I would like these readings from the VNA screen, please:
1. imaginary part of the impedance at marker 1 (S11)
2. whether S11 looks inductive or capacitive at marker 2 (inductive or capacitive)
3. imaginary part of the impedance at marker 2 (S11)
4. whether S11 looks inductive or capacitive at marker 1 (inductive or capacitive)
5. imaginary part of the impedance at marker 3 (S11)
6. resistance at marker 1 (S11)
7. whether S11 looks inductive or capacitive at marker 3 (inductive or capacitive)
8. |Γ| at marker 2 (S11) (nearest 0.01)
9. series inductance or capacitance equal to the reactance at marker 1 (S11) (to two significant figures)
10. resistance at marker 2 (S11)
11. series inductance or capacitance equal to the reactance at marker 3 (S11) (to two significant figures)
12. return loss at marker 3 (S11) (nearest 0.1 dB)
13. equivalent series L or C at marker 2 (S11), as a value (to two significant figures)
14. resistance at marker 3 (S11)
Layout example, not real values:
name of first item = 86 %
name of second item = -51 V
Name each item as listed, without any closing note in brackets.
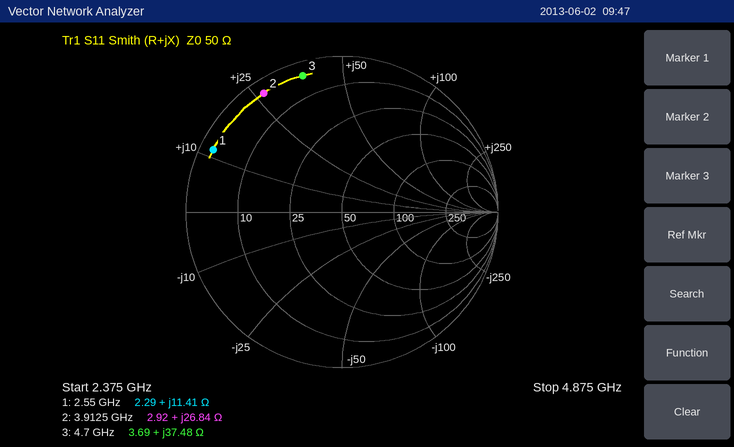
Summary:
imaginary part of the impedance at marker 1 = +11.41 Ω
whether S11 looks inductive or capacitive at marker 2 = inductive
imaginary part of the impedance at marker 2 = +26.84 Ω
whether S11 looks inductive or capacitive at marker 1 = inductive
imaginary part of the impedance at marker 3 = +37.48 Ω
resistance at marker 1 = 2.29 Ω
whether S11 looks inductive or capacitive at marker 3 = inductive
|Γ| at marker 2 (S11) = 0.91
series inductance or capacitance equal to the reactance at marker 1 (S11) = 710 pH
resistance at marker 2 = 2.92 Ω
series inductance or capacitance equal to the reactance at marker 3 (S11) = 1.3 nH
return loss at marker 3 (S11) = 0.8 dB
equivalent series L or C at marker 2 (S11), as a value = 1.1 nH
resistance at marker 3 = 3.69 Ω
